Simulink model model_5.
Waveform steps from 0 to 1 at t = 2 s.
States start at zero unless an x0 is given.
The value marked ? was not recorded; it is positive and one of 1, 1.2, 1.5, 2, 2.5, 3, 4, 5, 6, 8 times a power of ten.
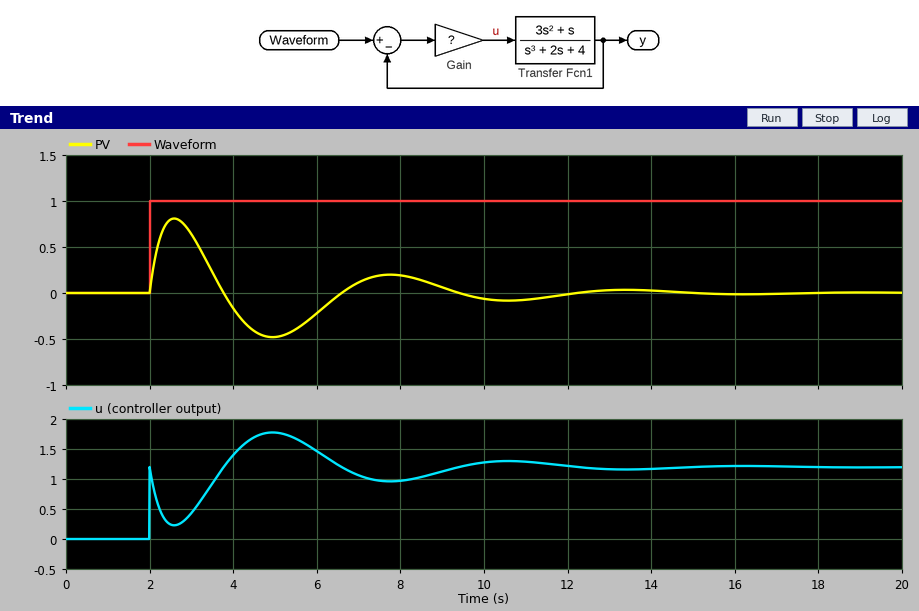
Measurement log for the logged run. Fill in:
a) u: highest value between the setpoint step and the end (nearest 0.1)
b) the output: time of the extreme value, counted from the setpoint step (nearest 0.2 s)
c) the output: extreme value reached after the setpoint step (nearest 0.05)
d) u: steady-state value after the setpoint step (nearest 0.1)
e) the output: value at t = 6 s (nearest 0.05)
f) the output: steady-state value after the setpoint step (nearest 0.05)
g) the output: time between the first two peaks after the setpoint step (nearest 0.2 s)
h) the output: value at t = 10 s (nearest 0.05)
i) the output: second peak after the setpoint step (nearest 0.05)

1.8
0.6 s
0.80
1.2
-0.20
0.00
5.2 s
-0.05
0.20
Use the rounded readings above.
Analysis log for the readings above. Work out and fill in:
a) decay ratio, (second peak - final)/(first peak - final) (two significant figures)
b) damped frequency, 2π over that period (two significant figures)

0.25
1.2 rad/s
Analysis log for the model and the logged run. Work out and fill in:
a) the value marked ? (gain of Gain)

1.2
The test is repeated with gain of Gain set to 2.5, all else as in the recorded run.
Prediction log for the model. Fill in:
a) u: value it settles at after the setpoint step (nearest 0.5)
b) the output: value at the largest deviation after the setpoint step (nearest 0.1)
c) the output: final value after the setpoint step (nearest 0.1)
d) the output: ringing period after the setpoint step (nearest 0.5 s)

2.5
0.9
0.0
8.0 s
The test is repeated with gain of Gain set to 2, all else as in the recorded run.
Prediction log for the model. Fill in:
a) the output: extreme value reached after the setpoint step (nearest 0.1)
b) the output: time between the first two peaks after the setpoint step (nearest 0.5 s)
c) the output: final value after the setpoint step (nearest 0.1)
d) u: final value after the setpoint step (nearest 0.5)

0.9
7.0 s
0.0
2.0
